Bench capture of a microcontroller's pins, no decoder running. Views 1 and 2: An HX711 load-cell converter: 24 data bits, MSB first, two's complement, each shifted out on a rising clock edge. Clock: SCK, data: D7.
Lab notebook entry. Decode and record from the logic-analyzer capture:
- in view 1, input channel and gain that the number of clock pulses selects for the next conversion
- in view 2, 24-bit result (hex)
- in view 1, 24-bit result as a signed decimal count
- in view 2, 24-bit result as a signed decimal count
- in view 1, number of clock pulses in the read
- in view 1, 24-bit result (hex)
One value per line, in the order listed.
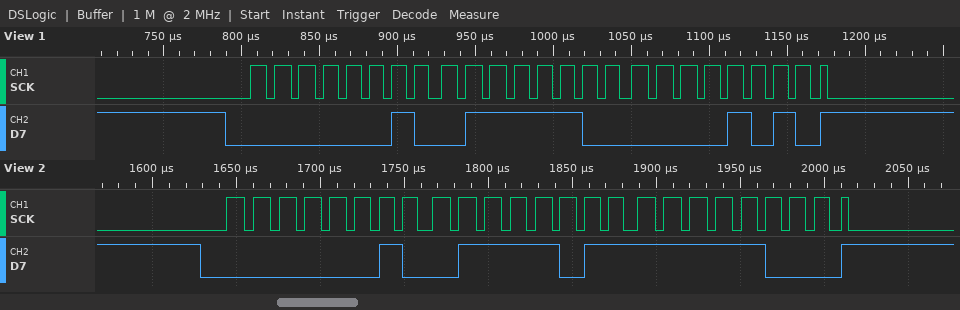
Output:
channel A, gain 128
0x027BF8
162826
162808
25
0x027C0A
